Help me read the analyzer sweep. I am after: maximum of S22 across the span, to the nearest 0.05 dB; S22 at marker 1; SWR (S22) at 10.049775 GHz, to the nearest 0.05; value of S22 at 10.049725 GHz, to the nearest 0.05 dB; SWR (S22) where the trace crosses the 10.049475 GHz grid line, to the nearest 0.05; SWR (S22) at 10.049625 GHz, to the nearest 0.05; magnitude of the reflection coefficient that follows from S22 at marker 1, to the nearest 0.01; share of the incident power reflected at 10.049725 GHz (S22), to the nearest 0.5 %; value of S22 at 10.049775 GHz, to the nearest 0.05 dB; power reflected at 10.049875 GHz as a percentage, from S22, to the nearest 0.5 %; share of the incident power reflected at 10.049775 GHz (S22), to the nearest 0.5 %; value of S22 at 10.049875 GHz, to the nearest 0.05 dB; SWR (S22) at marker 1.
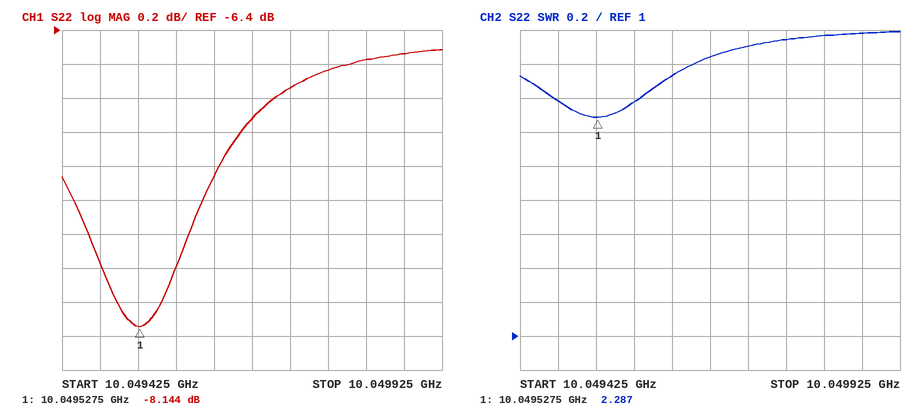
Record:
-6.50 dB
-8.144 dB
2.75
-6.75 dB
2.40
2.55
0.39
21.0 %
-6.65 dB
22.0 %
21.5 %
-6.55 dB
2.287
